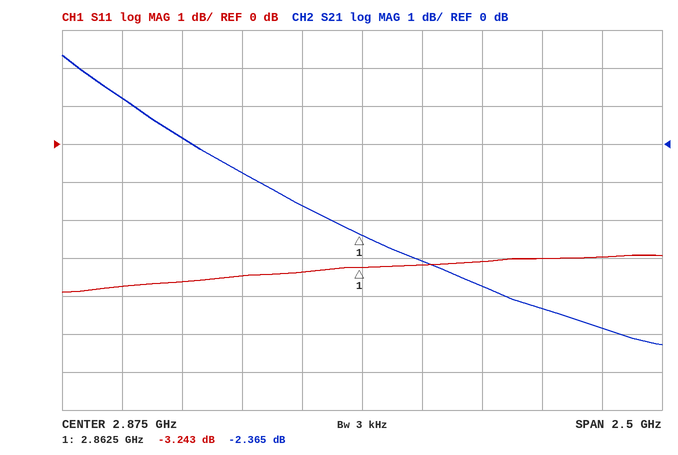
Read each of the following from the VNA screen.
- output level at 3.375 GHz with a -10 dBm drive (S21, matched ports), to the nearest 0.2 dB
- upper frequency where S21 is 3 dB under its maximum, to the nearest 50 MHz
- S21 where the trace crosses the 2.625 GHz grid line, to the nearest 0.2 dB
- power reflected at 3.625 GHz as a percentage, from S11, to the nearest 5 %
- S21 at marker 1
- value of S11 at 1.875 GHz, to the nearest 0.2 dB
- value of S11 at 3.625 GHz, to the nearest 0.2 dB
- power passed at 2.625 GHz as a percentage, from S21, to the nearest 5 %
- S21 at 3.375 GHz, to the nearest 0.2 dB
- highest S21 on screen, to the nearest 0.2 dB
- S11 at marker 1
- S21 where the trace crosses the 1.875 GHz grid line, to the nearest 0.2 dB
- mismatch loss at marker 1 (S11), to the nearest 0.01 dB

-13.8 dBm
2.35 GHz
-1.6 dB
50 %
-2.365 dB
-3.8 dB
-3.0 dB
70 %
-3.8 dB
2.4 dB
-3.243 dB
1.2 dB
2.79 dB
